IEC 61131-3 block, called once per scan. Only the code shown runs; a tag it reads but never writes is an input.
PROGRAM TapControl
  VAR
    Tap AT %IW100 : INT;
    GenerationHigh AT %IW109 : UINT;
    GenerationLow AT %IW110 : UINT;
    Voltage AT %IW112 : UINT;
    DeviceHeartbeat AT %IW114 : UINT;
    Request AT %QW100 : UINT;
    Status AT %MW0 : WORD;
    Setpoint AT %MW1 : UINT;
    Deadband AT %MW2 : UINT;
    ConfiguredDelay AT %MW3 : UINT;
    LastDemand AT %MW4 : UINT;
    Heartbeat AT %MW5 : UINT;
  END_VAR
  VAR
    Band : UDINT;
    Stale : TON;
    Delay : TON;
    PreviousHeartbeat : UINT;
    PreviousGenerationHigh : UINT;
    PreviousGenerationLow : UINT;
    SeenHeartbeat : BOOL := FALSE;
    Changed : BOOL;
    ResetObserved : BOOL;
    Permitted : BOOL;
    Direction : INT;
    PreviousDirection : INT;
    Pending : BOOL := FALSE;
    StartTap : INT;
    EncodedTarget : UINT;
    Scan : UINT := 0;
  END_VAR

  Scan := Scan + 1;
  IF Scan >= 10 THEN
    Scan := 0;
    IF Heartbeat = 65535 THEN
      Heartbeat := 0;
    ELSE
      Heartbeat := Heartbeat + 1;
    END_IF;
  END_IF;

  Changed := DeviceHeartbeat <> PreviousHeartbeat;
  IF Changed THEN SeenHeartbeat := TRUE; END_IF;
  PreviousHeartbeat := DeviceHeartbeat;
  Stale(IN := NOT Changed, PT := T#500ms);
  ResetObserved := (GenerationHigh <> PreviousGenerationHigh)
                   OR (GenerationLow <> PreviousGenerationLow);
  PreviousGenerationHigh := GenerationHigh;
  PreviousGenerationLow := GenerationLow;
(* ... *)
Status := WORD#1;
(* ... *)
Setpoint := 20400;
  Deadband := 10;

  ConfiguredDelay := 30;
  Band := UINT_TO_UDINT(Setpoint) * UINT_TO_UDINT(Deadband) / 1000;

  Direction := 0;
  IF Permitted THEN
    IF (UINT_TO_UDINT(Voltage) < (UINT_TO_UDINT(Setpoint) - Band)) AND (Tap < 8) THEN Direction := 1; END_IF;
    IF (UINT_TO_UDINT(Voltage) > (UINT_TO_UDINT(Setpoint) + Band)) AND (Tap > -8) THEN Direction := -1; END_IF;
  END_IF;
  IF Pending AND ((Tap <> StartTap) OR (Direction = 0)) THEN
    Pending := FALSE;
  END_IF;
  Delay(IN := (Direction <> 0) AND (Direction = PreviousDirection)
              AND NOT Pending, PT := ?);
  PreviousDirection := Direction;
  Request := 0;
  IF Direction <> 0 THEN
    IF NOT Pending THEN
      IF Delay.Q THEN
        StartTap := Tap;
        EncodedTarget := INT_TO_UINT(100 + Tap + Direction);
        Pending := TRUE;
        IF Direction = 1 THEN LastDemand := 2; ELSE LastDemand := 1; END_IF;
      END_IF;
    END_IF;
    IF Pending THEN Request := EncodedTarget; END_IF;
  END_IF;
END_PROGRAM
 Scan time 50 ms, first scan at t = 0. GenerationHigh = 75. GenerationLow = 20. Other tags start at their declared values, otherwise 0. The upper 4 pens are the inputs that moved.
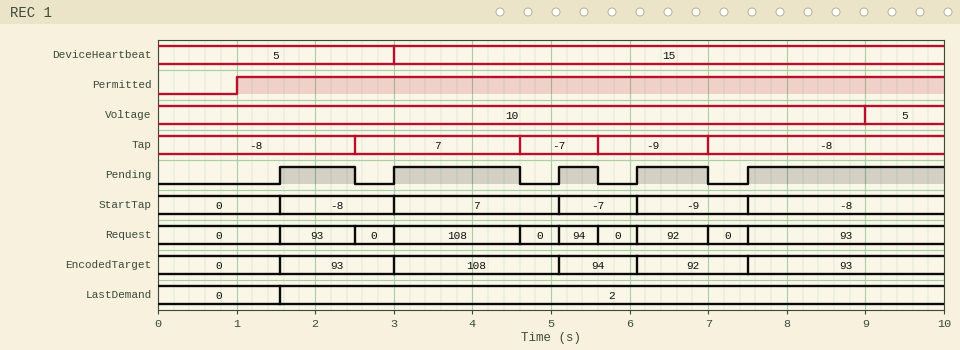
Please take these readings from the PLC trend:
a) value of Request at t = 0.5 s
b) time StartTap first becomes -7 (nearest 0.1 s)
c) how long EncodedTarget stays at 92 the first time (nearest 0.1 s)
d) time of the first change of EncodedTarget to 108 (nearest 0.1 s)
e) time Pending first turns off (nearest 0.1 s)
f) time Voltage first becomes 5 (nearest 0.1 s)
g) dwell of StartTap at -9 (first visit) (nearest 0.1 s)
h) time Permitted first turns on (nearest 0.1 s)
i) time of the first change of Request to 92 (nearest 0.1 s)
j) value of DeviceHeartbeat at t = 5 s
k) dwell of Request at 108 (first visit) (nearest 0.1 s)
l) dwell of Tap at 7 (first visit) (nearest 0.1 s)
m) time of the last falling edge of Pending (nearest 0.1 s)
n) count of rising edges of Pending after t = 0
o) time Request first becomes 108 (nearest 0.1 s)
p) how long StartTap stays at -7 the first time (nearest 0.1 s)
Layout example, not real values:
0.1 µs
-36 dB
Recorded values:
0
5.1 s
1.4 s
3.0 s
2.5 s
9.0 s
1.4 s
1.0 s
6.1 s
15
1.6 s
2.1 s
7.0 s
5
3.0 s
1.0 s
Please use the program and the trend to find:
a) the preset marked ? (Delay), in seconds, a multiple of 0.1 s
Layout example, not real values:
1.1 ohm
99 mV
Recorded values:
0.5 s
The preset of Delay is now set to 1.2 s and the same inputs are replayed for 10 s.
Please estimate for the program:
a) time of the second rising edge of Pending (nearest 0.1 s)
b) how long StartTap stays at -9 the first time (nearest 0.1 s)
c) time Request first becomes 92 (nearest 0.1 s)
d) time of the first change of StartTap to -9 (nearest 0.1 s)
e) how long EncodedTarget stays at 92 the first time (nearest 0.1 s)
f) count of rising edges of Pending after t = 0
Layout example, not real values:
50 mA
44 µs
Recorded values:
3.7 s
2.4 s
5.8 s
5.8 s
2.4 s
4
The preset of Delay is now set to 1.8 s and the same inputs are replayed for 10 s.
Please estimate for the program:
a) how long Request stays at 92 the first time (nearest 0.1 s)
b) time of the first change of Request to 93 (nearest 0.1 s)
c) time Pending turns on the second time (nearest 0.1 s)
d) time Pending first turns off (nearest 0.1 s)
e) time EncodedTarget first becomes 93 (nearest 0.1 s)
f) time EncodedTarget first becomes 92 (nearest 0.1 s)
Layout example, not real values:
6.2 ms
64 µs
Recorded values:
0.6 s
8.8 s
6.4 s
4.6 s
8.8 s
6.4 s
